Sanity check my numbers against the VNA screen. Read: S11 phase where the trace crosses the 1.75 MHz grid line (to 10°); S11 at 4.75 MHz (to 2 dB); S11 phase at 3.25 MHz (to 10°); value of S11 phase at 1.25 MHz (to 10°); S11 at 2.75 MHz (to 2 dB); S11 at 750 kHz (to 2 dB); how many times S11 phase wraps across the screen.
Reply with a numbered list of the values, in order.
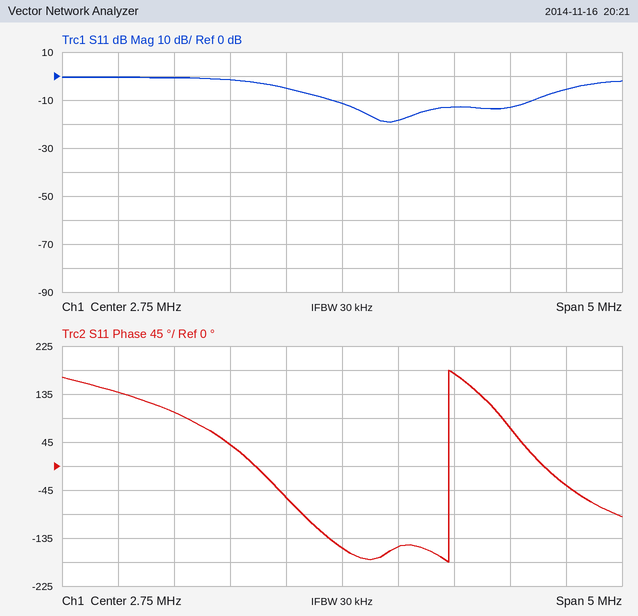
1. 40°
2. -6 dB
3. -150°
4. 100°
5. -12 dB
6. 0 dB
7. 1
